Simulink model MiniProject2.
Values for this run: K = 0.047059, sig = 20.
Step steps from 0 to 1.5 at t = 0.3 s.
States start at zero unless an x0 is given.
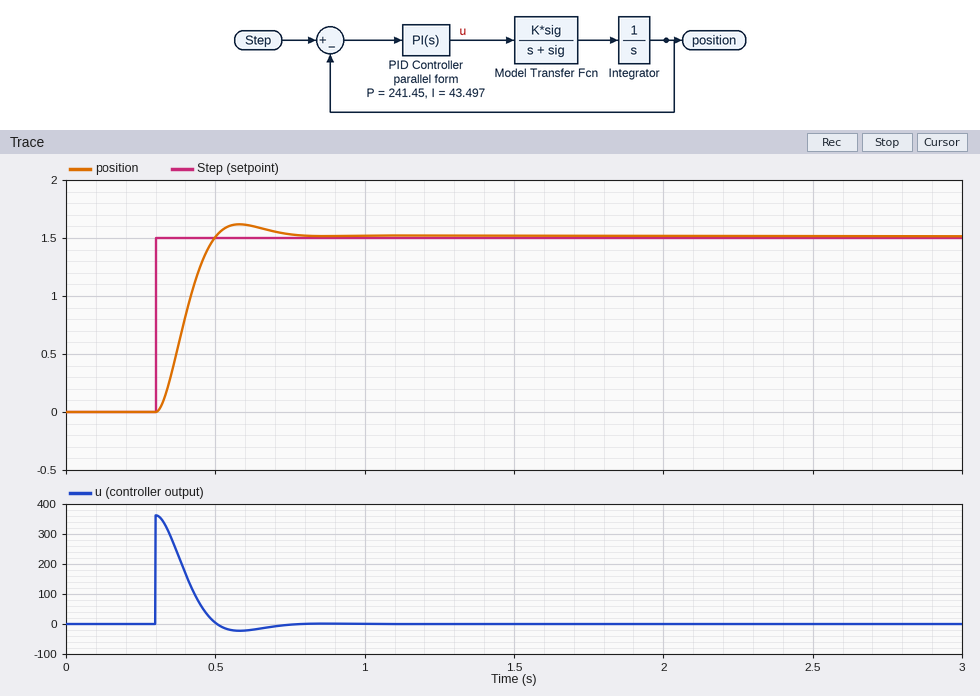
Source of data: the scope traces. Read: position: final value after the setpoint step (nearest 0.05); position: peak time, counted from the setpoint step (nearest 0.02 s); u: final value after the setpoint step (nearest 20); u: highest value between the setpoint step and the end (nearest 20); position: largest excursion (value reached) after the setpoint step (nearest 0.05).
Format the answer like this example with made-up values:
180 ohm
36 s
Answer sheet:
1.50
0.28 s
0
360
1.60
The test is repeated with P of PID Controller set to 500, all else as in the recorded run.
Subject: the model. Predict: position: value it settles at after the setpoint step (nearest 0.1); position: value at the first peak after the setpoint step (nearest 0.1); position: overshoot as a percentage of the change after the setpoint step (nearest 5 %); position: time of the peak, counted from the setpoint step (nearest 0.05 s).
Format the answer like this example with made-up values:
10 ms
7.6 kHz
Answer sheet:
1.5
1.8
20 %
0.15 s
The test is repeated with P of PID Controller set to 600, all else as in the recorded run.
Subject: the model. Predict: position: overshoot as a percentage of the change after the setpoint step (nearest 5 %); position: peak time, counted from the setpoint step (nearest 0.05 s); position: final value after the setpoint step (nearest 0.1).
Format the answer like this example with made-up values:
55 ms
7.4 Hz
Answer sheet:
25 %
0.15 s
1.5
